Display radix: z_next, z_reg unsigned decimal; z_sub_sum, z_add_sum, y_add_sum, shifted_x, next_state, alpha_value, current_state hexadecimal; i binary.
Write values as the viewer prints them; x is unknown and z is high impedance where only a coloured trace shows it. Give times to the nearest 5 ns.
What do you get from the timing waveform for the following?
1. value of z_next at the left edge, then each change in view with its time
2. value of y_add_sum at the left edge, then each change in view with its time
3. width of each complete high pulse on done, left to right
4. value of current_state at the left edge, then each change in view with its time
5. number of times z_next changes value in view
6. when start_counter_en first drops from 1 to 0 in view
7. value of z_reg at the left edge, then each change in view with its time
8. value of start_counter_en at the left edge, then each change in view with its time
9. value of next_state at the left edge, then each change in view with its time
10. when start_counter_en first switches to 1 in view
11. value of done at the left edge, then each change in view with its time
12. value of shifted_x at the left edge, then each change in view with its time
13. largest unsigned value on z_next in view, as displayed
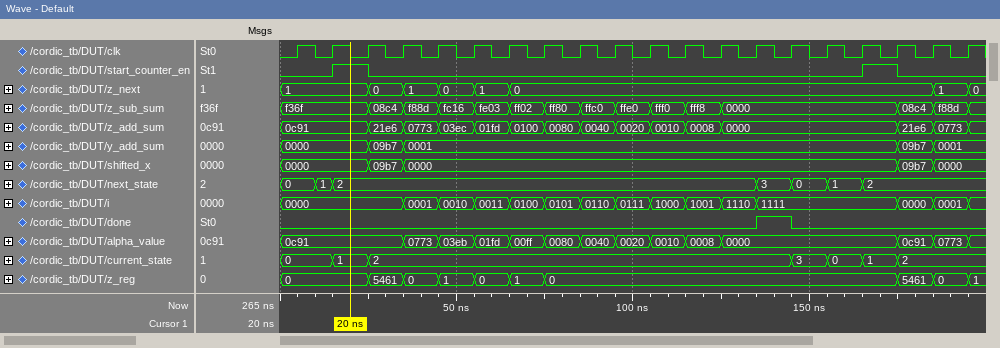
1, 0 at 25 ns, 1 at 35 ns, 0 at 45 ns, 1 at 55 ns, 0 at 65 ns, 1 at 185 ns, 0 at 195 ns
0000, 09b7 at 25 ns, 0001 at 35 ns, 09b7 at 175 ns, 0001 at 185 ns
10 ns
0, 1 at 15 ns, 2 at 25 ns, 3 at 145 ns, 0 at 155 ns, 1 at 165 ns, 2 at 175 ns
7
25 ns
0, 5461 at 25 ns, 0 at 35 ns, 1 at 45 ns, 0 at 55 ns, 1 at 65 ns, 0 at 75 ns, 5461 at 175 ns, 0 at 185 ns, 1 at 195 ns
0, 1 at 15 ns, 0 at 25 ns, 1 at 165 ns, 0 at 175 ns
0, 1 at 10 ns, 2 at 15 ns, 3 at 135 ns, 0 at 145 ns, 1 at 155 ns, 2 at 165 ns
15 ns
0, 1 at 135 ns, 0 at 145 ns
0000, 09b7 at 25 ns, 0000 at 35 ns, 09b7 at 175 ns, 0000 at 185 ns
1
